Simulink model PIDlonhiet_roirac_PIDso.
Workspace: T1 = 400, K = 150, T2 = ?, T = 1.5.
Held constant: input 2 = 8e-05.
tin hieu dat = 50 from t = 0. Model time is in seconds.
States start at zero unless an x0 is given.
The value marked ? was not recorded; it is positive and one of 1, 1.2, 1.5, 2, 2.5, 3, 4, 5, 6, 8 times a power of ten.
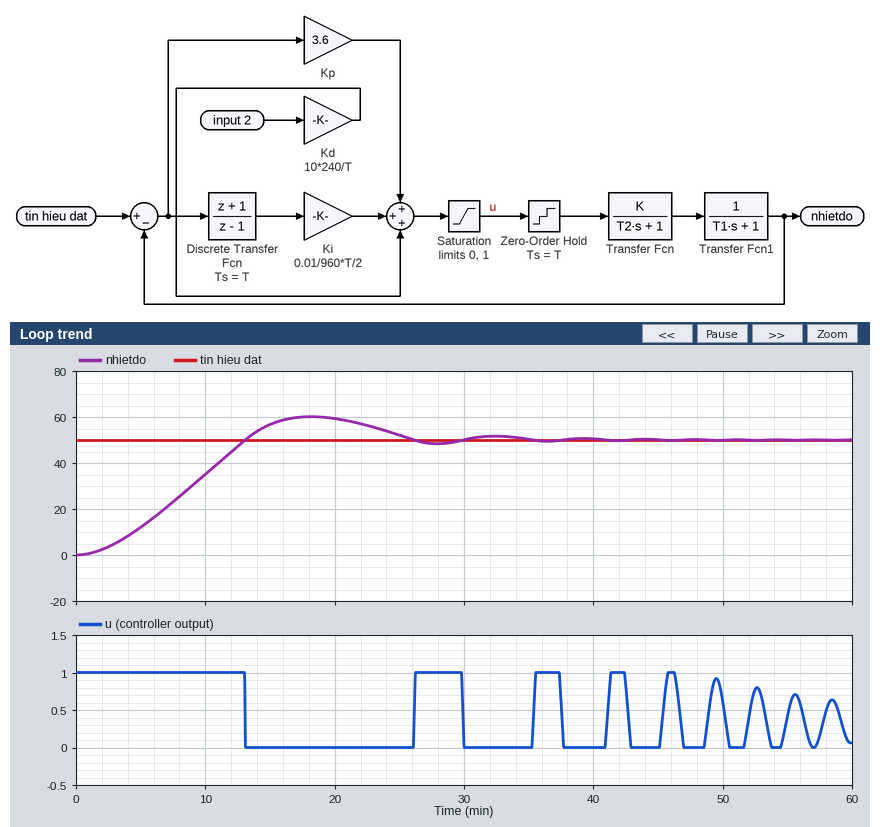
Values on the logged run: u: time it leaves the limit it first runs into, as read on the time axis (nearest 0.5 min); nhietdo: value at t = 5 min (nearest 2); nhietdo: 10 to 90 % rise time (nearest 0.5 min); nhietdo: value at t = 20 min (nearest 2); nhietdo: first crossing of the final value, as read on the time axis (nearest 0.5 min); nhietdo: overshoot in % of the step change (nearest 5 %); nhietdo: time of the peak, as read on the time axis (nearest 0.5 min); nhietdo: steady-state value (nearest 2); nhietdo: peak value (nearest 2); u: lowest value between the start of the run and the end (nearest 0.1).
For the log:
13.0 min
12
9.0 min
60
13.0 min
20 %
18.0 min
50
60
0.0
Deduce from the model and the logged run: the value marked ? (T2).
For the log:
1000
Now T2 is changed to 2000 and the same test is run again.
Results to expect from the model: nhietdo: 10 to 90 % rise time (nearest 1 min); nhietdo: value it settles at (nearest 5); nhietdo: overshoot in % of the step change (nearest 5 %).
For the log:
14 min
50
15 %
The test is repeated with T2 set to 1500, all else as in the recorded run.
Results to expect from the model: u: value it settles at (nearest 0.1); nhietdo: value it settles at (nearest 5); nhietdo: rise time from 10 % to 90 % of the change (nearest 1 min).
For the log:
0.3
50
12 min
